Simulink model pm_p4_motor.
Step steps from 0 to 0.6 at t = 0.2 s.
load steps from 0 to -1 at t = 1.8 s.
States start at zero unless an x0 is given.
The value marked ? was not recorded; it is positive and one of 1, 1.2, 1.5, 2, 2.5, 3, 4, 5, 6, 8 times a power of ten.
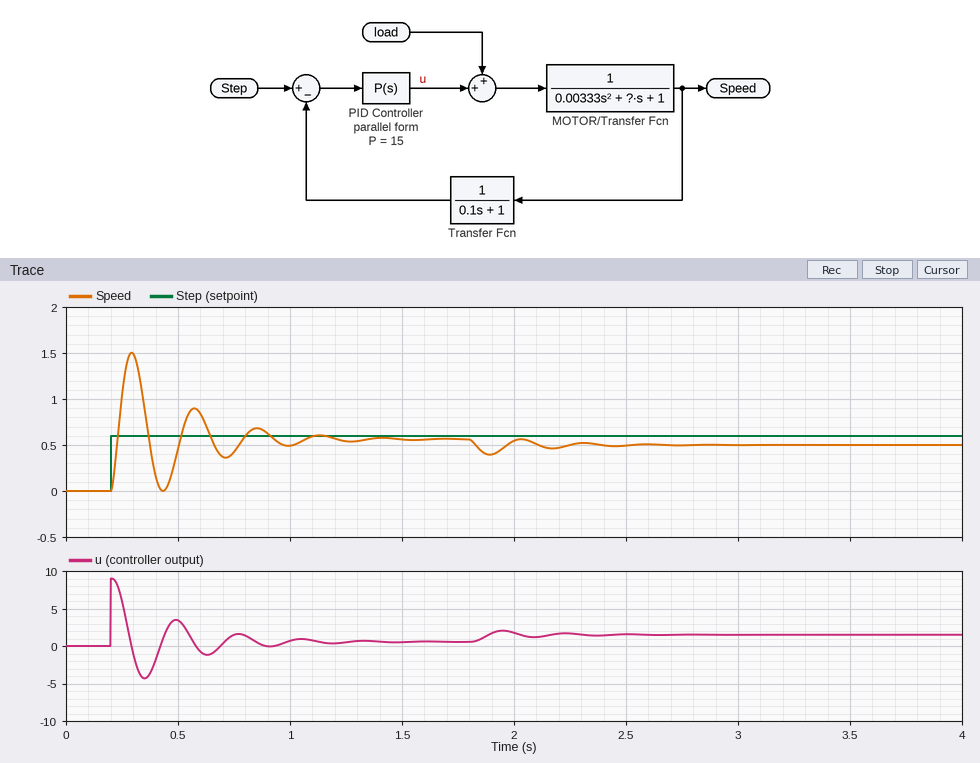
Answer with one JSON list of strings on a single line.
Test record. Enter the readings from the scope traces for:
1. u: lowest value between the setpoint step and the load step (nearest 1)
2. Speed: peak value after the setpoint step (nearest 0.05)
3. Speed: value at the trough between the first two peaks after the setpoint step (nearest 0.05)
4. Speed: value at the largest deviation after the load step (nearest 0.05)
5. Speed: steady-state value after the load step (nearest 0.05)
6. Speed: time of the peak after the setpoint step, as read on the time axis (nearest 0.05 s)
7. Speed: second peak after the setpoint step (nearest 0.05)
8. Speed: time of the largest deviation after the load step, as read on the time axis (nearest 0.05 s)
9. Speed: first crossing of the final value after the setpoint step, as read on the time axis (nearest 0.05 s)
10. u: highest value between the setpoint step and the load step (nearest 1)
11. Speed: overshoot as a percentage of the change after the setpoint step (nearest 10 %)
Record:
["-4", "1.50", "0.00", "0.40", "0.50", "0.30 s", "0.90", "1.90 s", "0.25 s", "9", "170 %"]
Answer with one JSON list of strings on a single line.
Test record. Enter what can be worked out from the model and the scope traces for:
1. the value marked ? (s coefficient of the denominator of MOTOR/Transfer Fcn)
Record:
["0.3"]
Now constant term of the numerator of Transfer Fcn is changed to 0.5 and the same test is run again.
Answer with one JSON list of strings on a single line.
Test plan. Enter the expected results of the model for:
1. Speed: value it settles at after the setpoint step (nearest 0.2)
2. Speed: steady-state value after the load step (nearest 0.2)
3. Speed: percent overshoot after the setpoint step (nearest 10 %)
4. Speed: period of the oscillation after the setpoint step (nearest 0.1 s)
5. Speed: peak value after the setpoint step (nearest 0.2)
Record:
["1.0", "1.0", "90 %", "0.4 s", "2.0"]
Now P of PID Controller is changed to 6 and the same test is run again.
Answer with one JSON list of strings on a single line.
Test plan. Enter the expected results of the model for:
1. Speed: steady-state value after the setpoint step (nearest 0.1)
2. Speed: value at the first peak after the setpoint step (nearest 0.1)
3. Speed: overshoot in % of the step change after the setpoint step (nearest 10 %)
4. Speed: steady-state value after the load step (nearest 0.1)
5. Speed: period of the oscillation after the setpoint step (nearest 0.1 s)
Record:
["0.5", "0.9", "70 %", "0.4", "0.4 s"]
